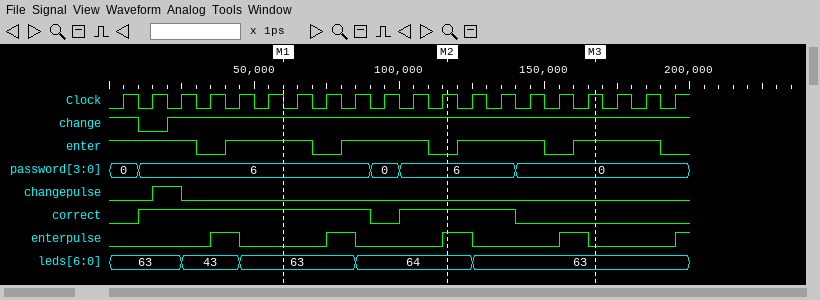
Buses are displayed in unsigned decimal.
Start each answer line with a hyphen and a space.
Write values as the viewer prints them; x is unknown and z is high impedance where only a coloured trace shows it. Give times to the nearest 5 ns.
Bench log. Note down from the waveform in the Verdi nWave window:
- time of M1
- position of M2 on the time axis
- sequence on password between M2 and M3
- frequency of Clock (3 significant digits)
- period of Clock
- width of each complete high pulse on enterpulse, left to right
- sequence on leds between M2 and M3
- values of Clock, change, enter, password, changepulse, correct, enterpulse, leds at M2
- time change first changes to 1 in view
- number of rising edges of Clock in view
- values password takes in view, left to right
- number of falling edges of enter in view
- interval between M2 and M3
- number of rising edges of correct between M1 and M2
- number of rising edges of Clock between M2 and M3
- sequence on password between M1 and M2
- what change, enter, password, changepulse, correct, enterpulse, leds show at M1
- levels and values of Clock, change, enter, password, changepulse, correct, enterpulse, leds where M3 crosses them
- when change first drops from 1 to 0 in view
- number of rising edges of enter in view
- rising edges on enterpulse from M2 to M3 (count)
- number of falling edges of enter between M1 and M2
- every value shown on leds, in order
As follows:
- 60 ns
- 115 ns
- 6, 0
- 100 MHz
- 10 ns
- 10 ns, 10 ns, 10 ns, 10 ns
- 64, 63
- Clock=1, change=1, enter=0, password=6, changepulse=0, correct=1, enterpulse=1, leds=64
- 20 ns
- 20
- 0, 6, 0, 6, 0
- 5
- 50 ns
- 1
- 5
- 6, 0, 6
- change=1, enter=1, password=6, changepulse=0, correct=1, enterpulse=0, leds=63
- Clock=1, change=1, enter=1, password=0, changepulse=0, correct=0, enterpulse=0, leds=63
- 10 ns
- 4
- 1
- 2
- 63, 43, 63, 64, 63
